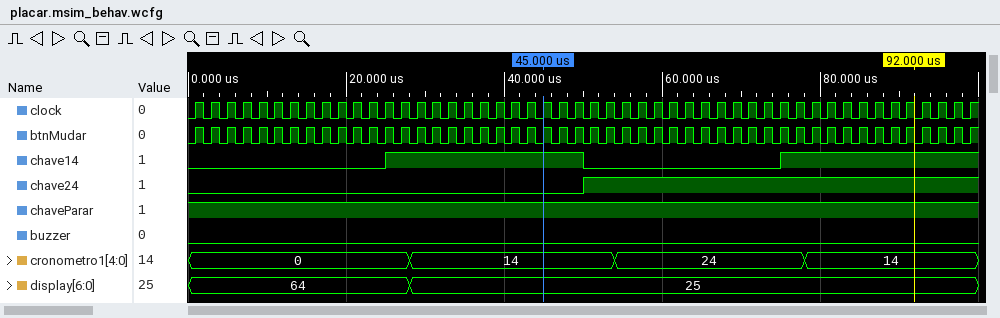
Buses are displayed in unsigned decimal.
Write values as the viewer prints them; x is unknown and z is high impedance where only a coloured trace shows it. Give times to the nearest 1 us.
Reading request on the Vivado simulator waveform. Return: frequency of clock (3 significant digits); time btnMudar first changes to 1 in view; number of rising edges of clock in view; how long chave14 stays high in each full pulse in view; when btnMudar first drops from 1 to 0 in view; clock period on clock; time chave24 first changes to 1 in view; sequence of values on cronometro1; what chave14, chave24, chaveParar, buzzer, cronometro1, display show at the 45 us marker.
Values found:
500 kHz
1 us
50
25 us
2 us
2 us
50 us
0, 14, 24, 14
chave14=1, chave24=0, chaveParar=1, buzzer=0, cronometro1=14, display=25
